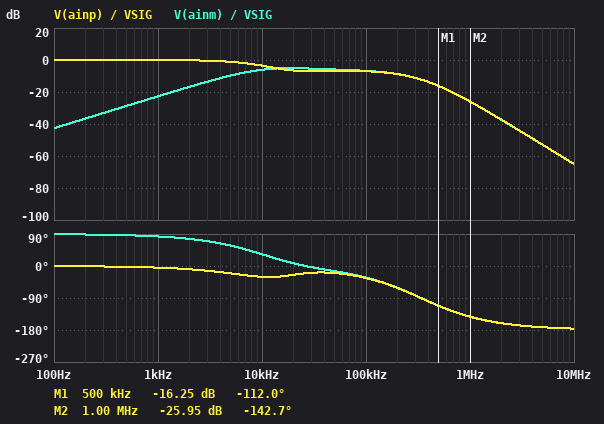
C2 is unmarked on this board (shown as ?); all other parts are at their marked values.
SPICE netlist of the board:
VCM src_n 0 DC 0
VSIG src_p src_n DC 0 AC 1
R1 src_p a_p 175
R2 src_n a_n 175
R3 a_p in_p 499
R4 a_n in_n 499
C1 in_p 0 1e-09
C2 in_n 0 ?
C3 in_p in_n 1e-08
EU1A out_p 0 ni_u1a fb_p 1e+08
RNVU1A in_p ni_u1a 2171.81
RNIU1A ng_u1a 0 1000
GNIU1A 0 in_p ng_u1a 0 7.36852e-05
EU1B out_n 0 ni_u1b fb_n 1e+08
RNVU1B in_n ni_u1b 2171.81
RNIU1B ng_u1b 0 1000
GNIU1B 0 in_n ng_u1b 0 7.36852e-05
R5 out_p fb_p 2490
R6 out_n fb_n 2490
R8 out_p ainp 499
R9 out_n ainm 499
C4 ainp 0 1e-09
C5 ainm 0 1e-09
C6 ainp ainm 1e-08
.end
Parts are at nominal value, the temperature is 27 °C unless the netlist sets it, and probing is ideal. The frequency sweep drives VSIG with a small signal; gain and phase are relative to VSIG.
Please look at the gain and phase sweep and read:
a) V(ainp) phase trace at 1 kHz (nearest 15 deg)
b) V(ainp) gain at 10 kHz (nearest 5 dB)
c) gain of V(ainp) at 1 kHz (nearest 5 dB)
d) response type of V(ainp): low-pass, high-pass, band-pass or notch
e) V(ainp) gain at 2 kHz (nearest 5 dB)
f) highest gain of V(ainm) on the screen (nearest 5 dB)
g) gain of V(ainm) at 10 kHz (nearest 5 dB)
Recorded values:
0 deg
-5 dB
0 dB
low-pass
0 dB
-5 dB
-5 dB
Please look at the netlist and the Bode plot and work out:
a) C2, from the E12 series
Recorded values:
330 pF
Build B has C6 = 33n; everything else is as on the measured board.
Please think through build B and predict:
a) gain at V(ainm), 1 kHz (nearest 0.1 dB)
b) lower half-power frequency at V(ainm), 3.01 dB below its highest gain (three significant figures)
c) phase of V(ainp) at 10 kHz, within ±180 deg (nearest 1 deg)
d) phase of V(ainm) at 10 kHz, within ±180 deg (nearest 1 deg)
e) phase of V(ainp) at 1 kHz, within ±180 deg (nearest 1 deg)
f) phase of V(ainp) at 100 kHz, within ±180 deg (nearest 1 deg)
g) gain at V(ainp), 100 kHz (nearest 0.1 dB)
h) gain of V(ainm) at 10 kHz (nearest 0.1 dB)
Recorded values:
-16.9 dB
3.36 kHz
-23 deg
13 deg
-9 deg
-33 deg
-6.9 dB
-5.1 dB
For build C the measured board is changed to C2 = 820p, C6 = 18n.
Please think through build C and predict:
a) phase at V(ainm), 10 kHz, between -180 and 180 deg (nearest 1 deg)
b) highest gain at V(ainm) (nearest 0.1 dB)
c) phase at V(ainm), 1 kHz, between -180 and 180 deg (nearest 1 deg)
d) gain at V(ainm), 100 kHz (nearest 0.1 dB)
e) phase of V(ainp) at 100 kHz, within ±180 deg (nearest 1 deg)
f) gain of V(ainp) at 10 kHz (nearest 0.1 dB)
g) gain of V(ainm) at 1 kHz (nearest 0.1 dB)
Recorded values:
23 deg
-5.0 dB
81 deg
-7.0 dB
-39 deg
-4.9 dB
-20.2 dB
